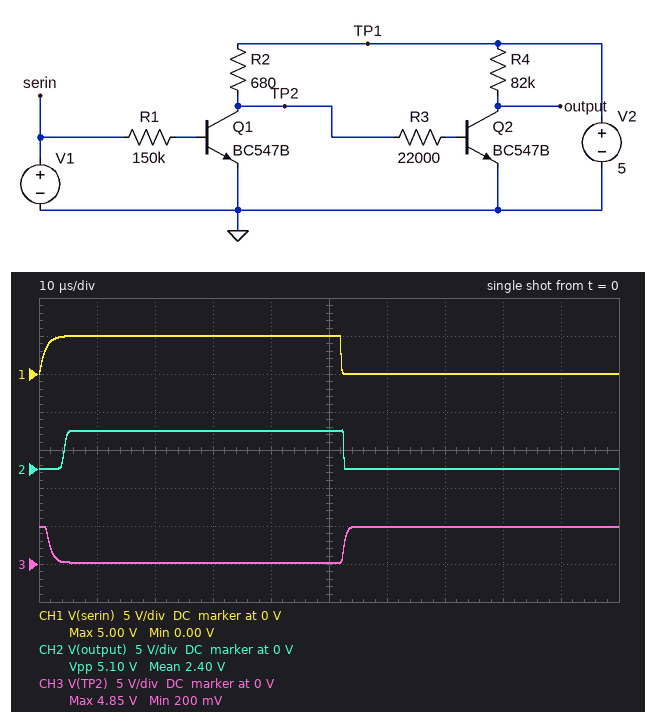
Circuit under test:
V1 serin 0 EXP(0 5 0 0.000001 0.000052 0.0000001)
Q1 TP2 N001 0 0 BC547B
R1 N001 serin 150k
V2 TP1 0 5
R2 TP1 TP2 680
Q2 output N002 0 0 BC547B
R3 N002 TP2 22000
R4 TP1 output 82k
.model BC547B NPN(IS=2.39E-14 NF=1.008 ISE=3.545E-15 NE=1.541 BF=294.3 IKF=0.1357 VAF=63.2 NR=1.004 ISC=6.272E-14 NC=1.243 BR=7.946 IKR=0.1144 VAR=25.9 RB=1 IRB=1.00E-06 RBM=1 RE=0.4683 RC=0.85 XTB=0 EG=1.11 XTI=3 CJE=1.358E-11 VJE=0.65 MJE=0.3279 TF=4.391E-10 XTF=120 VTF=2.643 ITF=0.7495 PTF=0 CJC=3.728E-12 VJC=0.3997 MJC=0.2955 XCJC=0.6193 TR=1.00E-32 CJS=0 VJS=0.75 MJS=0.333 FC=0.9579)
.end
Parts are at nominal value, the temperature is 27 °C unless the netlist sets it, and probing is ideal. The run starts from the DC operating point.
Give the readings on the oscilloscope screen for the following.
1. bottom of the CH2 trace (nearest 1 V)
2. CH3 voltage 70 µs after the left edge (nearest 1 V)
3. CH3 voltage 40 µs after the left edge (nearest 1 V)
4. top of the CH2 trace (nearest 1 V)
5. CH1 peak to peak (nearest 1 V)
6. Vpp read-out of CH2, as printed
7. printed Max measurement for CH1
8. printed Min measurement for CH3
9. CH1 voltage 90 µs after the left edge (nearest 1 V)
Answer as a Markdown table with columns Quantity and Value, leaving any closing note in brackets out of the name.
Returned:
| Quantity | Value |
|---|---|
| bottom of the CH2 trace | 0 V |
| CH3 voltage 70 µs after the left edge | 5 V |
| CH3 voltage 40 µs after the left edge | 0 V |
| top of the CH2 trace | 5 V |
| CH1 peak to peak | 5 V |
| Vpp read-out of CH2, as printed | 5.10 V |
| printed Max measurement for CH1 | 5.00 V |
| printed Min measurement for CH3 | 200 mV |
| CH1 voltage 90 µs after the left edge | 0 V |
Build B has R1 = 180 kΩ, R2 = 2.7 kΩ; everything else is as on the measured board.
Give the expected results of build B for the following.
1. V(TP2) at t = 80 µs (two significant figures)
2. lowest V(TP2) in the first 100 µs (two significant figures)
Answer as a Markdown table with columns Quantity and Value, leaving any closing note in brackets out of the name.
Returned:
| Quantity | Value |
|---|---|
| V(TP2) at t = 80 µs | 4.5 V |
| lowest V(TP2) in the first 100 µs | 82 mV |
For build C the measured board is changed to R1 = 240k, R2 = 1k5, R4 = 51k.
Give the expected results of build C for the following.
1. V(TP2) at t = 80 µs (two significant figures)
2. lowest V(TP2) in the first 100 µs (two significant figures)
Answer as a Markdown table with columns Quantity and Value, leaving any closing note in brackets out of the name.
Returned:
| Quantity | Value |
|---|---|
| V(TP2) at t = 80 µs | 4.7 V |
| lowest V(TP2) in the first 100 µs | 130 mV |
